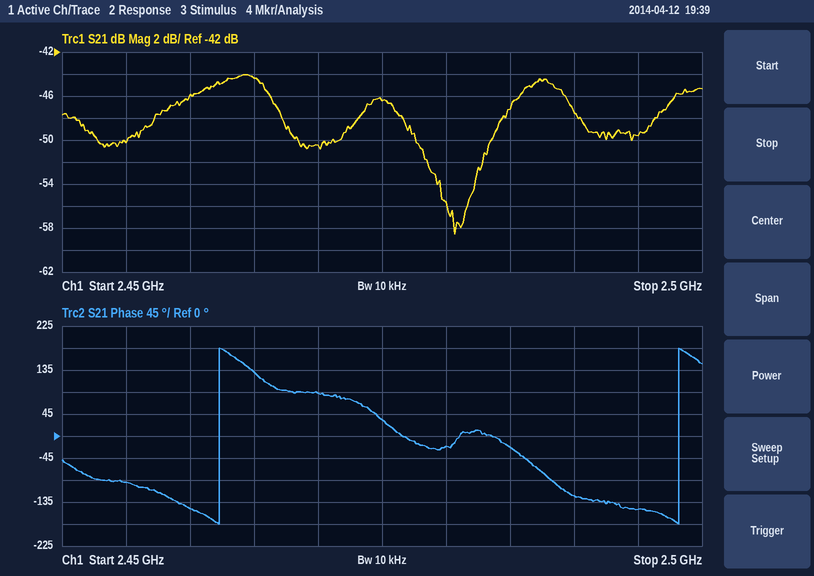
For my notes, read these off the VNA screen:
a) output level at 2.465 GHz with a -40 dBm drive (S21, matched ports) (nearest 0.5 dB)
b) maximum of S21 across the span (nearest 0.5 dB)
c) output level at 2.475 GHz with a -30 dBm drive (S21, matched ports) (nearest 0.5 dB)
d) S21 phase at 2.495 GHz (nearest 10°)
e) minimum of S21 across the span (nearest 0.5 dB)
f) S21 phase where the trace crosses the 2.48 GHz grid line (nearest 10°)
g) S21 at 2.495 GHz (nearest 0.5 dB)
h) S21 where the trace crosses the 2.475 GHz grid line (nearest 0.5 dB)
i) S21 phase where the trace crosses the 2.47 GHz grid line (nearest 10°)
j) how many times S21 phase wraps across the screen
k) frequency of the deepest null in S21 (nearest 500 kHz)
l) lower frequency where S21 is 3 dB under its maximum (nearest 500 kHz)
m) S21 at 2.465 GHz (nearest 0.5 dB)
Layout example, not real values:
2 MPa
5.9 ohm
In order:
-84.5 dBm
-44.0 dB
-76.5 dBm
-150°
-58.5 dB
-20°
-49.5 dB
-46.5 dB
90°
2
2.4805 GHz
2.4585 GHz
-44.5 dB
